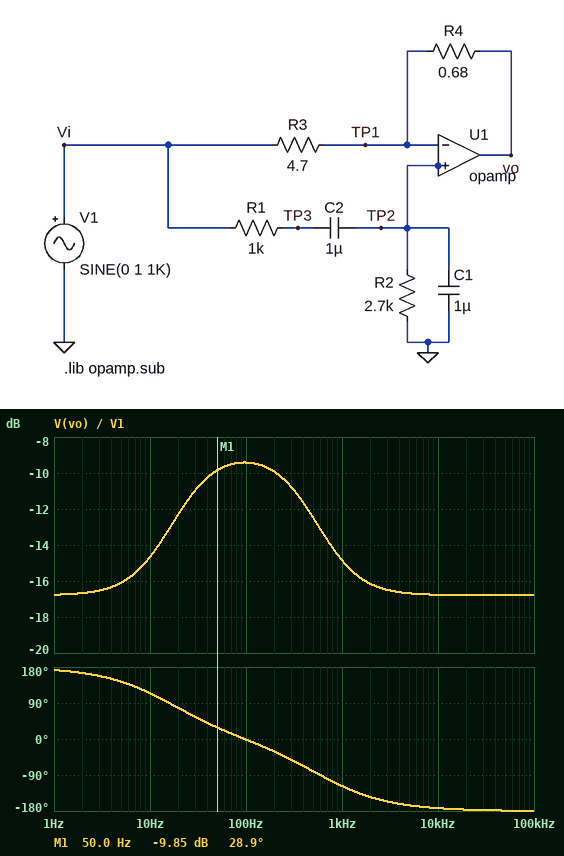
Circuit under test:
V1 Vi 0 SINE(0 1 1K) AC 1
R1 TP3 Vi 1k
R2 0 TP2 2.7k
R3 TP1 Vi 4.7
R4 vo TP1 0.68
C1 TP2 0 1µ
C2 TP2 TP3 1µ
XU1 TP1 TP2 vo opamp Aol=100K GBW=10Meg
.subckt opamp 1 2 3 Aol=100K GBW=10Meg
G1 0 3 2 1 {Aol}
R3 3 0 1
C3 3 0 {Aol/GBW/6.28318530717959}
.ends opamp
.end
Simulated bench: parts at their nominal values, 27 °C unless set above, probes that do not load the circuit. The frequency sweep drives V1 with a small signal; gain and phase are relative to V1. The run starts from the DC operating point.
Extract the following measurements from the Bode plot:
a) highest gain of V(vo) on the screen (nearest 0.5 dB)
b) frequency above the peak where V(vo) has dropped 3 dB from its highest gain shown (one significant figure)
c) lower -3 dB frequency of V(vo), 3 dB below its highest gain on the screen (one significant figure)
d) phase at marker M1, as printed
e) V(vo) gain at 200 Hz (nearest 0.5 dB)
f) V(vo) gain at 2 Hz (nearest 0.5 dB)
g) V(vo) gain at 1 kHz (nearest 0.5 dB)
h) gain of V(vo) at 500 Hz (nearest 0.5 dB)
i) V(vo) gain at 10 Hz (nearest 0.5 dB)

-9.5 dB
500 Hz
20 Hz
28.9 deg
-10.0 dB
-16.5 dB
-15.0 dB
-12.5 dB
-14.5 dB
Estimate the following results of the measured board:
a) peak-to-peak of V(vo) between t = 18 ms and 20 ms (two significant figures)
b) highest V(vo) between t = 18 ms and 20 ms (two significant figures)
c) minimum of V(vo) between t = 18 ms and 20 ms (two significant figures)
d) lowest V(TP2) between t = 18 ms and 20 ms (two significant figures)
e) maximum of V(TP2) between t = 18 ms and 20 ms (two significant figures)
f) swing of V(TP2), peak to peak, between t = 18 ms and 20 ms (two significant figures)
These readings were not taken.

360 mV
180 mV
-180 mV
-150 mV
150 mV
300 mV
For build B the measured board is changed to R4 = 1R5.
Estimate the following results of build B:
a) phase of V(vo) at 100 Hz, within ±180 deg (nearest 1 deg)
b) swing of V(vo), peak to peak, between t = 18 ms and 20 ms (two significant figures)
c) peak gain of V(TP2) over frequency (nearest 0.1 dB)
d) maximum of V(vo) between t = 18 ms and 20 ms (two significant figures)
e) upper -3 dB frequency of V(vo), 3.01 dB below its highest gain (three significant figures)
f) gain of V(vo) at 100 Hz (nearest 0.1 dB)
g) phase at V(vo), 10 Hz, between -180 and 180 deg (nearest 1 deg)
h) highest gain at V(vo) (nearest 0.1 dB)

-2 deg
620 mV
-7.5 dB
310 mV
7.58 MHz
-12.5 dB
141 deg
-9.9 dB
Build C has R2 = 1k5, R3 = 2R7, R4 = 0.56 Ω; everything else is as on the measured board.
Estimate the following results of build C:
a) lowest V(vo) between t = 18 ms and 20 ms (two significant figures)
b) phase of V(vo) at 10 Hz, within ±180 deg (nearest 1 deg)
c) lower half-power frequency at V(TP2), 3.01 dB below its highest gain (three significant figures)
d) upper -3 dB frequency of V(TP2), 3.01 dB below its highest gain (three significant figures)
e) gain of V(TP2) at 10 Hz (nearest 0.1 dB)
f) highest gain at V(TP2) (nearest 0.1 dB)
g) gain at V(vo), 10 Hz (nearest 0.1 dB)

-210 mV
149 deg
36.6 Hz
461 Hz
-20.7 dB
-8.5 dB
-13.6 dB
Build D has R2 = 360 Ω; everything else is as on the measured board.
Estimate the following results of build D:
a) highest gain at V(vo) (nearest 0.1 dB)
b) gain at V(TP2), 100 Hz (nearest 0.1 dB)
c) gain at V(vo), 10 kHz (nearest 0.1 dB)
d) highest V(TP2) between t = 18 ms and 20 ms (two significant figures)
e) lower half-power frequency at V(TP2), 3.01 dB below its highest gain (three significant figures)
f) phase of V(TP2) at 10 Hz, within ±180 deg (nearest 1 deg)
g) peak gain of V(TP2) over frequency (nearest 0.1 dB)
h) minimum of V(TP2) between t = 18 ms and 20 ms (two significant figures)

-16.8 dB
-15.7 dB
-16.8 dB
130 mV
83.4 Hz
84 deg
-13.6 dB
-130 mV
